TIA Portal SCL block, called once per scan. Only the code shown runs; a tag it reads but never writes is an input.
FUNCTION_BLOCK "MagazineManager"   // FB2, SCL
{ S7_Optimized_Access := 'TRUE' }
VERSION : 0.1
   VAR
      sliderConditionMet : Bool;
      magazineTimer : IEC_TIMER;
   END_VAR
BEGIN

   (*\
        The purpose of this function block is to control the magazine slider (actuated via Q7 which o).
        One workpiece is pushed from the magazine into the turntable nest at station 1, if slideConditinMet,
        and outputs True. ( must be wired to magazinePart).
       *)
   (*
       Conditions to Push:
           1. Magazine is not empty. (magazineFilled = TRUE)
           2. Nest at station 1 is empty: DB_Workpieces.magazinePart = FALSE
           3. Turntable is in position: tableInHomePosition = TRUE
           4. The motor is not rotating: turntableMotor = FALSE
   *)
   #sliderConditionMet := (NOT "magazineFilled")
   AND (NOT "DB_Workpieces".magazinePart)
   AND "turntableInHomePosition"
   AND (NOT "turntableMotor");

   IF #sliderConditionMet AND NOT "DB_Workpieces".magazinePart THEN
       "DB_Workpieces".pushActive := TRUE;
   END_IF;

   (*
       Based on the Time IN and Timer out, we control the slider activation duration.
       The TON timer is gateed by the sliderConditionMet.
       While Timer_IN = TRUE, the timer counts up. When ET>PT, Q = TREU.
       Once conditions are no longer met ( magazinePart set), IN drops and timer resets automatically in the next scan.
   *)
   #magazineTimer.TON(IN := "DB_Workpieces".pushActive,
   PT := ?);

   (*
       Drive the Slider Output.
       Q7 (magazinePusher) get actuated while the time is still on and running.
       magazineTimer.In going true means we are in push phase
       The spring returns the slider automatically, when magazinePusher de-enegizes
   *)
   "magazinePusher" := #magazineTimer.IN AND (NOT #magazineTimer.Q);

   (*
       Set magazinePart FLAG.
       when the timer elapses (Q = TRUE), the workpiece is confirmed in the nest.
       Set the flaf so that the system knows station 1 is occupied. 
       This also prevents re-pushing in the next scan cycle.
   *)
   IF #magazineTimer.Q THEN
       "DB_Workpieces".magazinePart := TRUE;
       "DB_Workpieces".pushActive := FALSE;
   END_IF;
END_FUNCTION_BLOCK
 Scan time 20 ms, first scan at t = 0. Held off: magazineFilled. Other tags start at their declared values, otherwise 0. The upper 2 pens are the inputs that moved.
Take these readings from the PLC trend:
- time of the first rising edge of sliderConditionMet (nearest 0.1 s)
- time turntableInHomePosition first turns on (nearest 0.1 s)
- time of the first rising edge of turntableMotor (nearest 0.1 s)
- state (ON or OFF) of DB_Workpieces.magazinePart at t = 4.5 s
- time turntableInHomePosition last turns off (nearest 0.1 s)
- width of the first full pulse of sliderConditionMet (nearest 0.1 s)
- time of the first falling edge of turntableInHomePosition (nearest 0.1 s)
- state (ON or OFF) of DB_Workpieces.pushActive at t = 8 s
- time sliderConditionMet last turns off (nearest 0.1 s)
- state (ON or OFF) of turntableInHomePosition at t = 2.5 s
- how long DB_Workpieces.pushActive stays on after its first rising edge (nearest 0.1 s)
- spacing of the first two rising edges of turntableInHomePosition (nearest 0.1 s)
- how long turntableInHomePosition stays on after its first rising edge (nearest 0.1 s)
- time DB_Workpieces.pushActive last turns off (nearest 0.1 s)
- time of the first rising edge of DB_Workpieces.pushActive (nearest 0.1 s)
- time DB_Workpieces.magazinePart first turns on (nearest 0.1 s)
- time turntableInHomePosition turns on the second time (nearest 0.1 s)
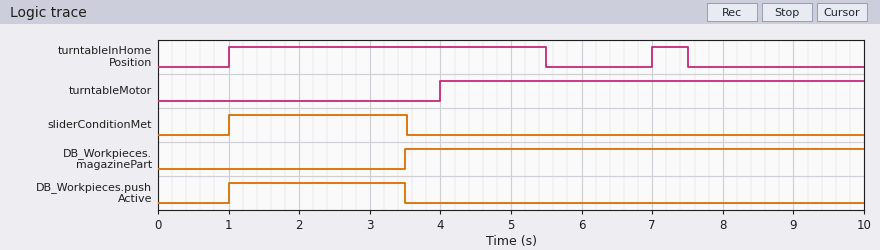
1.0 s
1.0 s
4.0 s
ON
7.5 s
2.5 s
5.5 s
OFF
3.5 s
ON
2.5 s
6.0 s
4.5 s
3.5 s
1.0 s
3.5 s
7.0 s
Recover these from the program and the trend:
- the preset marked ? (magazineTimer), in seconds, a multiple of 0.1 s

2.5 s
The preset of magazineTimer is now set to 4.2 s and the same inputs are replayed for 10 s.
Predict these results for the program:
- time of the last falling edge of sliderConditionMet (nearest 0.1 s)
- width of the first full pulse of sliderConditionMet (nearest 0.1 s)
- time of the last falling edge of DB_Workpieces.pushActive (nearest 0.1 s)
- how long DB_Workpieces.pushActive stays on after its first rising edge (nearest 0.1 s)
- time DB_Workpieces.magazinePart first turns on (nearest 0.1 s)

4.0 s
3.0 s
5.2 s
4.2 s
5.2 s
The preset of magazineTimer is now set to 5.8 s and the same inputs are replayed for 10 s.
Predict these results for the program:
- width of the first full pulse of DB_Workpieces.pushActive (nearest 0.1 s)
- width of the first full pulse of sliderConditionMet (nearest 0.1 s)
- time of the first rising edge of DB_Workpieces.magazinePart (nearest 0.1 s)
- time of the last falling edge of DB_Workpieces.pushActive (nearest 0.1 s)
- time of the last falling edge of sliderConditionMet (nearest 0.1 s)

5.8 s
3.0 s
6.8 s
6.8 s
4.0 s
